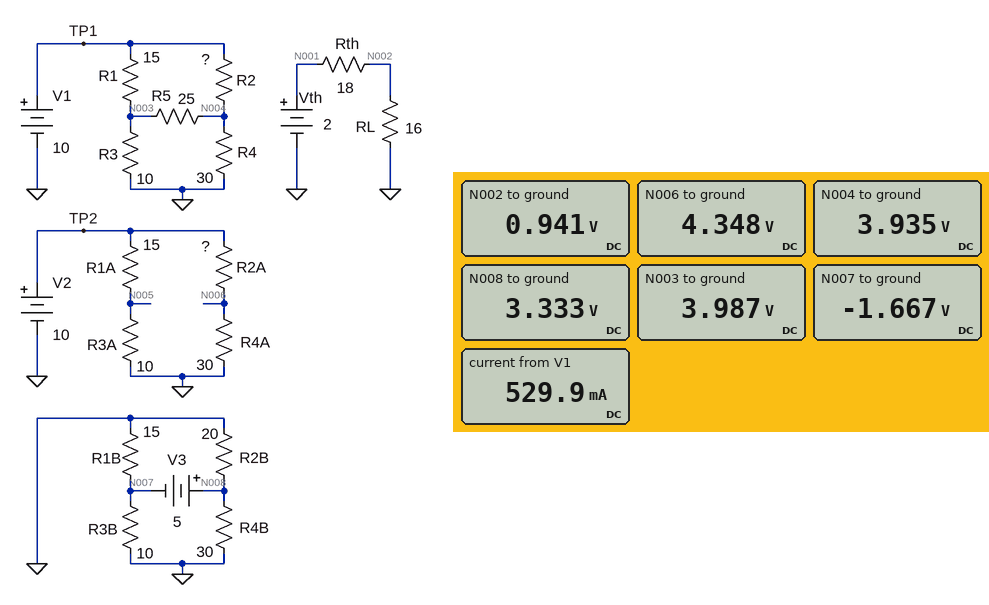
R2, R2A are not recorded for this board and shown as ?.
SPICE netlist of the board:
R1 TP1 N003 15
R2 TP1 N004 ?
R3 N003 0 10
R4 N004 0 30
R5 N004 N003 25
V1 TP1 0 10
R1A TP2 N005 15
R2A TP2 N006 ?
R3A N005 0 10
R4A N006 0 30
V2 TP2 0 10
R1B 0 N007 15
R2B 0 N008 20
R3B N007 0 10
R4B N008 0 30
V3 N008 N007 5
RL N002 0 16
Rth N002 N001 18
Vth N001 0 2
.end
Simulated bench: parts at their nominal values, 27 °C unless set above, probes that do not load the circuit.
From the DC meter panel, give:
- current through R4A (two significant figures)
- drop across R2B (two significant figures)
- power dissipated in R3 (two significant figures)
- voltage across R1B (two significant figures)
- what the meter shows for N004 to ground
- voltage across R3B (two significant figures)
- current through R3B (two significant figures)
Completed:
140 mA
3.3 V
1.6 W
1.7 V
3.935 V
1.7 V
170 mA
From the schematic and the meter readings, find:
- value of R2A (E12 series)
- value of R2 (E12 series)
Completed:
39 Ω
47 Ω
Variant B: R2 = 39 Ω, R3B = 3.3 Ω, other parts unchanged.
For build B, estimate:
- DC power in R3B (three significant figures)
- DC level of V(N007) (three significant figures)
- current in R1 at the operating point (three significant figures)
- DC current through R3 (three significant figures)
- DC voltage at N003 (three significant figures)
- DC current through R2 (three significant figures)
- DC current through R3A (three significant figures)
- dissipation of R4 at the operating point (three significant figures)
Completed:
256 mW
-920 mV
397 mA
404 mA
4.04 V
148 mA
400 mA
595 mW
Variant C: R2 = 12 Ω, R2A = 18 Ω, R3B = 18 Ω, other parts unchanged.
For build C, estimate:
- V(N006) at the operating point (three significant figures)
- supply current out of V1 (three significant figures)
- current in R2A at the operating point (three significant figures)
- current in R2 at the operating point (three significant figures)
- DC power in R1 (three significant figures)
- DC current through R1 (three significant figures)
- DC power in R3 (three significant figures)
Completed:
6.25 V
663 mA
208 mA
295 mA
2.03 W
368 mA
2.00 W
